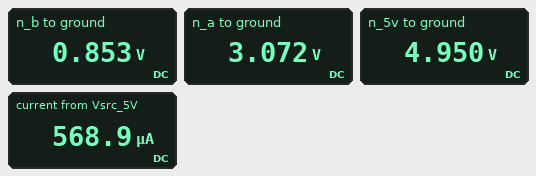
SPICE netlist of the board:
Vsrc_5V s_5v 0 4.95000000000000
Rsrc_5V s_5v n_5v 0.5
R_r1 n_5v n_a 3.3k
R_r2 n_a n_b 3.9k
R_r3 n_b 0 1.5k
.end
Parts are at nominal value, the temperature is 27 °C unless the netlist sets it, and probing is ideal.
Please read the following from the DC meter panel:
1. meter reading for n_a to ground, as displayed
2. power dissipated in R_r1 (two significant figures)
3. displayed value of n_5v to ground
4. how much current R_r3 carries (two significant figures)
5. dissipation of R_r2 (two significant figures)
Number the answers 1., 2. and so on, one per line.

1. 3.072 V
2. 1.1 mW
3. 4.950 V
4. 570 µA
5. 1.3 mW
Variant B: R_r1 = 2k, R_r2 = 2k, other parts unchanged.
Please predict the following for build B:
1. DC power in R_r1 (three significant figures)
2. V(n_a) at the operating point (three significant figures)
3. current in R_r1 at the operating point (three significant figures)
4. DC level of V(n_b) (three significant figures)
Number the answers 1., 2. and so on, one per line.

1. 1.62 mW
2. 3.15 V
3. 900 µA
4. 1.35 V
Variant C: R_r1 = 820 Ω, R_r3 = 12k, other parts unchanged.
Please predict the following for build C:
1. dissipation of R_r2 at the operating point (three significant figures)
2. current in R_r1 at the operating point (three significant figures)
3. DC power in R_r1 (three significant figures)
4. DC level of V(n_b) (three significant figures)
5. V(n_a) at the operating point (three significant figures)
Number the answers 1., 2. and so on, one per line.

1. 342 µW
2. 296 µA
3. 71.9 µW
4. 3.55 V
5. 4.71 V
